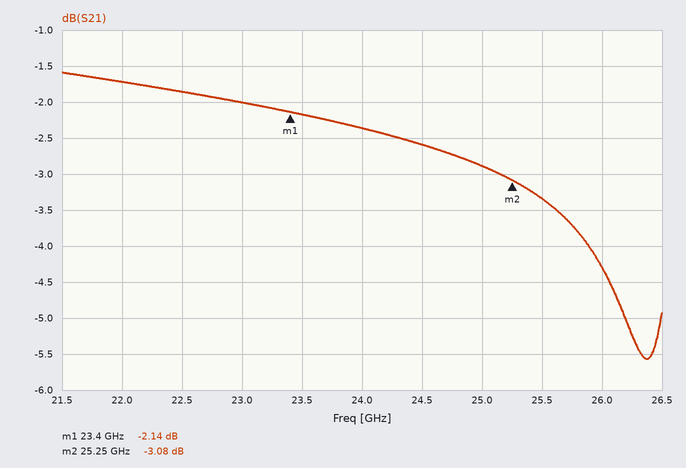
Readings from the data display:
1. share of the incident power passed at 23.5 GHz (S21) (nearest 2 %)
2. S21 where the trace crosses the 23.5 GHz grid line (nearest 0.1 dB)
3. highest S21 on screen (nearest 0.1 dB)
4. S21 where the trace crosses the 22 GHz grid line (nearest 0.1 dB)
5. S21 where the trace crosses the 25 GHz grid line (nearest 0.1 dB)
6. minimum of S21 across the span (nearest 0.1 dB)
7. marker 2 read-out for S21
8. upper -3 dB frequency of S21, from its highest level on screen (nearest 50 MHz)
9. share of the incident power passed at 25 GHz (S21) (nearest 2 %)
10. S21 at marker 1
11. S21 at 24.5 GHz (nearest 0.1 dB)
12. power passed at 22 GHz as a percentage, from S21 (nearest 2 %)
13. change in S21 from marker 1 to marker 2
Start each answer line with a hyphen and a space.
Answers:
- 60 %
- -2.2 dB
- -1.6 dB
- -1.7 dB
- -2.9 dB
- -5.6 dB
- -3.08 dB
- 26.10 GHz
- 52 %
- -2.14 dB
- -2.6 dB
- 68 %
- -0.94 dB
